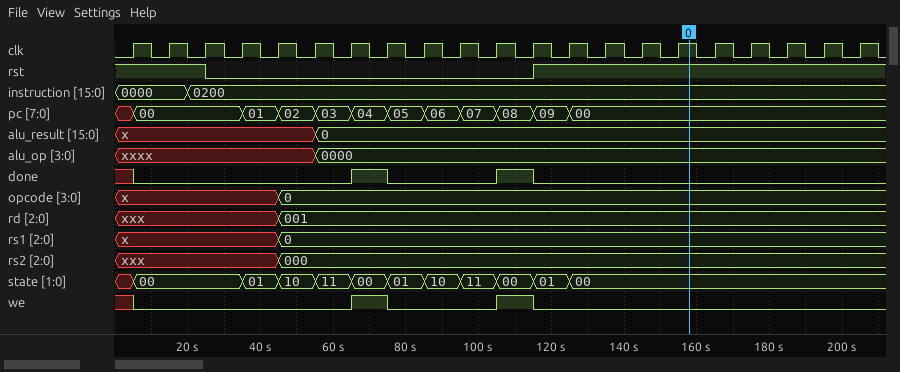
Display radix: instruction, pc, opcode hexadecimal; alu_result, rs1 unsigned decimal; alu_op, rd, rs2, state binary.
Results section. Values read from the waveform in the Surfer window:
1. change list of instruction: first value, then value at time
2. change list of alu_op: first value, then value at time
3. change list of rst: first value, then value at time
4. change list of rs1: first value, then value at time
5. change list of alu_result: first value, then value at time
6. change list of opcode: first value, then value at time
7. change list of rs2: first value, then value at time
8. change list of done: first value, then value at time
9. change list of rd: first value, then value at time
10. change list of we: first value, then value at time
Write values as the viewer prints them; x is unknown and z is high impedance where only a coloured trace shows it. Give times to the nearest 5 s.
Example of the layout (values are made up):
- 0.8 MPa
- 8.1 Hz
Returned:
- 0000, 0200 at 20 s
- xxxx, 0000 at 55 s
- 1, 0 at 25 s, 1 at 115 s
- x, 0 at 45 s
- x, 0 at 55 s
- x, 0 at 45 s
- xxx, 000 at 45 s
- x, 0 at 5 s, 1 at 65 s, 0 at 75 s, 1 at 105 s, 0 at 115 s
- xxx, 001 at 45 s
- x, 0 at 5 s, 1 at 65 s, 0 at 75 s, 1 at 105 s, 0 at 115 s
